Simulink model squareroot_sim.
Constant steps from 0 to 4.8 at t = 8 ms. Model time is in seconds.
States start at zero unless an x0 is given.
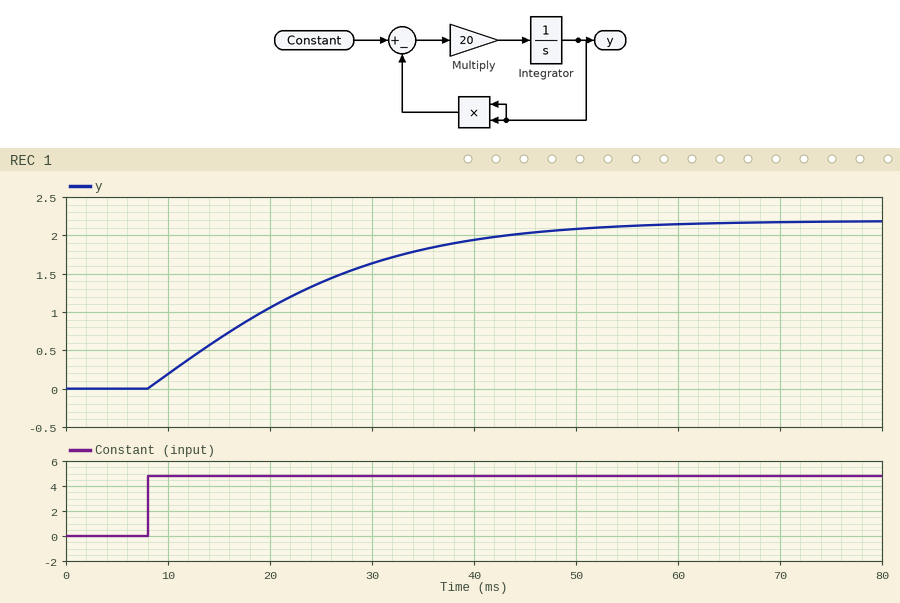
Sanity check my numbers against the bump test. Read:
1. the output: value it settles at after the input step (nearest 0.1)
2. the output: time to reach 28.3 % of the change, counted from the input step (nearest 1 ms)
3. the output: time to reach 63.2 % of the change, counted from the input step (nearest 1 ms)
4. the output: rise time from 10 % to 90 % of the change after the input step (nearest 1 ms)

2.2
7 ms
17 ms
31 ms
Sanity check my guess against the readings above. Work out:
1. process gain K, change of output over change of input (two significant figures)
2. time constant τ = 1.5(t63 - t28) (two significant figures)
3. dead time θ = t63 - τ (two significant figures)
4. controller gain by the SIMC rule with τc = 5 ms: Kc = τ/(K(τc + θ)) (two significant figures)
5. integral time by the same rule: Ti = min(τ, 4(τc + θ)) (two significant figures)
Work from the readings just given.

0.46
15 ms
2.0 ms
4.7
15 ms
